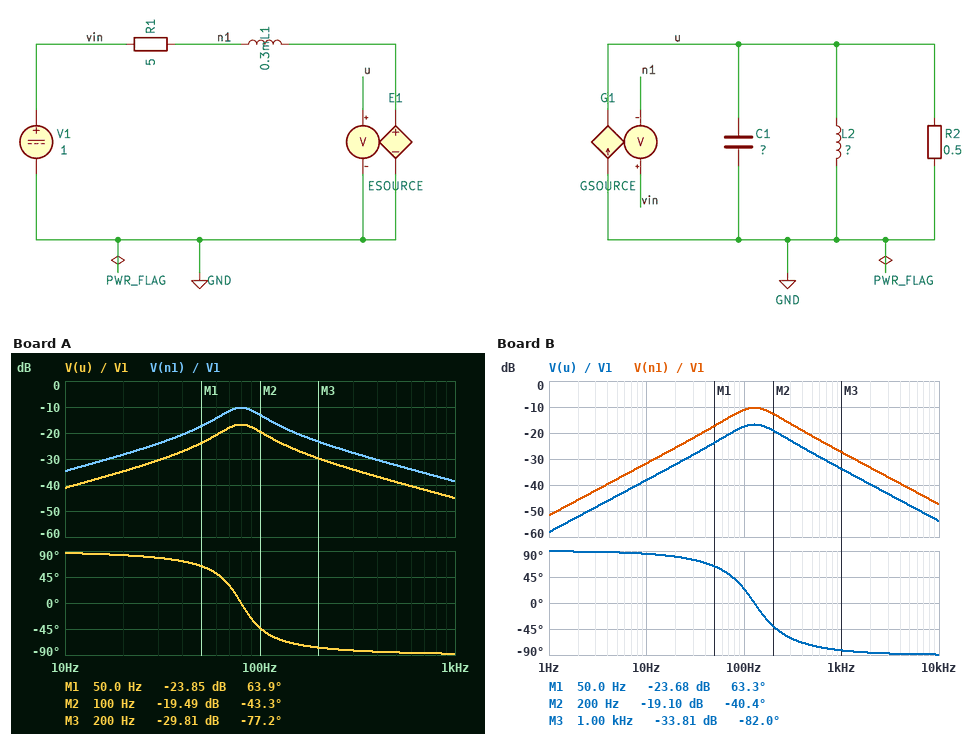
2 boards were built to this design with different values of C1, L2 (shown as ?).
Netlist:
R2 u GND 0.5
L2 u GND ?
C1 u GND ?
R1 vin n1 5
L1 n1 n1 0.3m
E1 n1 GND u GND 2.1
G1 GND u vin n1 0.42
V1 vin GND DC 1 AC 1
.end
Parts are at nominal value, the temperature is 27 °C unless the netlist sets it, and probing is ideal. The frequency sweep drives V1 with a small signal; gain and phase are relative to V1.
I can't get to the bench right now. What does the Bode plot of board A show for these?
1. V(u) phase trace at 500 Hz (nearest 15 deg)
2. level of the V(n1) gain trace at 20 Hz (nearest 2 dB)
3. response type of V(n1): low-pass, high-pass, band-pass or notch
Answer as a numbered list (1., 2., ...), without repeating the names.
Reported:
1. -90 deg
2. -28 dB
3. band-pass
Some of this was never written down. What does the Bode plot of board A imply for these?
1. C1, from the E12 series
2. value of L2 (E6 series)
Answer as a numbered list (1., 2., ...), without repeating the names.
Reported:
1. 12 mF
2. 330 µH
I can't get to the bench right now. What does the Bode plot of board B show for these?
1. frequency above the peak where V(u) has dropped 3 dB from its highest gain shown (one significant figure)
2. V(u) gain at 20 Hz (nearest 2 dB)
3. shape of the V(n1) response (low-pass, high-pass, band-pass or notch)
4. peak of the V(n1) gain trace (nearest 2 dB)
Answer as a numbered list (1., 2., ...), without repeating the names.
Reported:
1. 200 Hz
2. -32 dB
3. band-pass
4. -10 dB
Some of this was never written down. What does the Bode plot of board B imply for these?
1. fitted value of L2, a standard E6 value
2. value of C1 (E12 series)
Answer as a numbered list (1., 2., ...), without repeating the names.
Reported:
1. 470 µH
2. 3.3 mF
